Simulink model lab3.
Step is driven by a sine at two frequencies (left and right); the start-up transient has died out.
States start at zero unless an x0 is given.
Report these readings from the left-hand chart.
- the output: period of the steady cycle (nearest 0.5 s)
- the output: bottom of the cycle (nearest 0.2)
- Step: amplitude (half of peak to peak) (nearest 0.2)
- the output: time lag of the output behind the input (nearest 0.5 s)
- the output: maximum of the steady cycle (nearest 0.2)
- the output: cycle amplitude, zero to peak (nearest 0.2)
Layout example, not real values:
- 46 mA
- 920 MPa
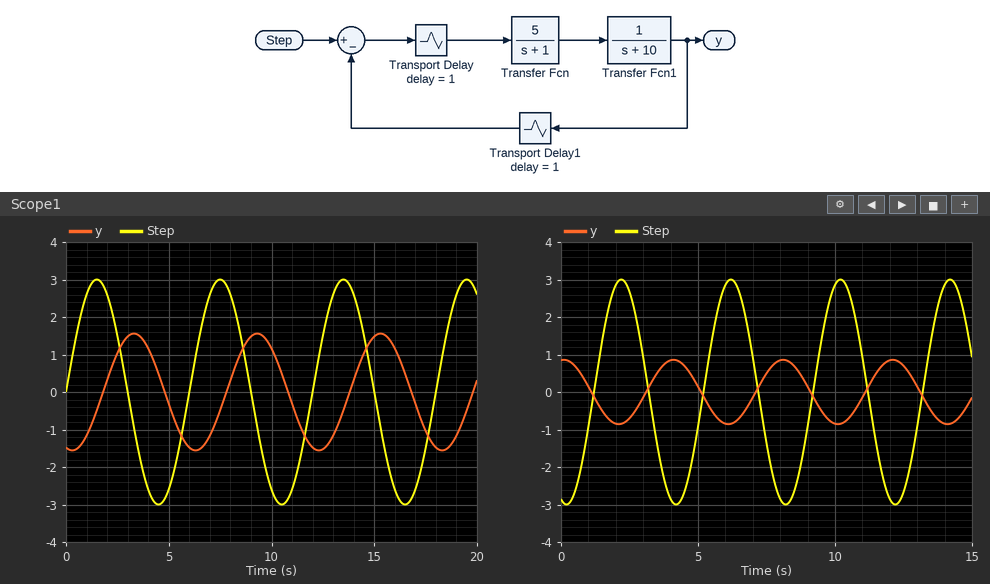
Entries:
- 6.0 s
- -1.6
- 3.0
- 2.0 s
- 1.6
- 1.6
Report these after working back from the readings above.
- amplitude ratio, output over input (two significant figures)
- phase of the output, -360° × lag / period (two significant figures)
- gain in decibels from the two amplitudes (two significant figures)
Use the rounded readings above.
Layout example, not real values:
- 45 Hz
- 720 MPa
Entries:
- 0.53
- -120°
- -5.5 dB
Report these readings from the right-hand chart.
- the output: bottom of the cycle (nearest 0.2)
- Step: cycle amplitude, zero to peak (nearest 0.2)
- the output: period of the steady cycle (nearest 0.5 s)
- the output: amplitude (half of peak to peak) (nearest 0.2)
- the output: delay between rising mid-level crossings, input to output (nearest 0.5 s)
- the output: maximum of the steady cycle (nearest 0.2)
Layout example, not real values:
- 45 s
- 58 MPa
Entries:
- -0.8
- 3.0
- 4.0 s
- 0.8
- 2.0 s
- 0.8
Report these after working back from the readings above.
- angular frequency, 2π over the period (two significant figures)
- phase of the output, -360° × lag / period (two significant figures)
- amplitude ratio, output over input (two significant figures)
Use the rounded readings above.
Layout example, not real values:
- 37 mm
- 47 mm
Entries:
- 1.6 rad/s
- -180°
- 0.27
